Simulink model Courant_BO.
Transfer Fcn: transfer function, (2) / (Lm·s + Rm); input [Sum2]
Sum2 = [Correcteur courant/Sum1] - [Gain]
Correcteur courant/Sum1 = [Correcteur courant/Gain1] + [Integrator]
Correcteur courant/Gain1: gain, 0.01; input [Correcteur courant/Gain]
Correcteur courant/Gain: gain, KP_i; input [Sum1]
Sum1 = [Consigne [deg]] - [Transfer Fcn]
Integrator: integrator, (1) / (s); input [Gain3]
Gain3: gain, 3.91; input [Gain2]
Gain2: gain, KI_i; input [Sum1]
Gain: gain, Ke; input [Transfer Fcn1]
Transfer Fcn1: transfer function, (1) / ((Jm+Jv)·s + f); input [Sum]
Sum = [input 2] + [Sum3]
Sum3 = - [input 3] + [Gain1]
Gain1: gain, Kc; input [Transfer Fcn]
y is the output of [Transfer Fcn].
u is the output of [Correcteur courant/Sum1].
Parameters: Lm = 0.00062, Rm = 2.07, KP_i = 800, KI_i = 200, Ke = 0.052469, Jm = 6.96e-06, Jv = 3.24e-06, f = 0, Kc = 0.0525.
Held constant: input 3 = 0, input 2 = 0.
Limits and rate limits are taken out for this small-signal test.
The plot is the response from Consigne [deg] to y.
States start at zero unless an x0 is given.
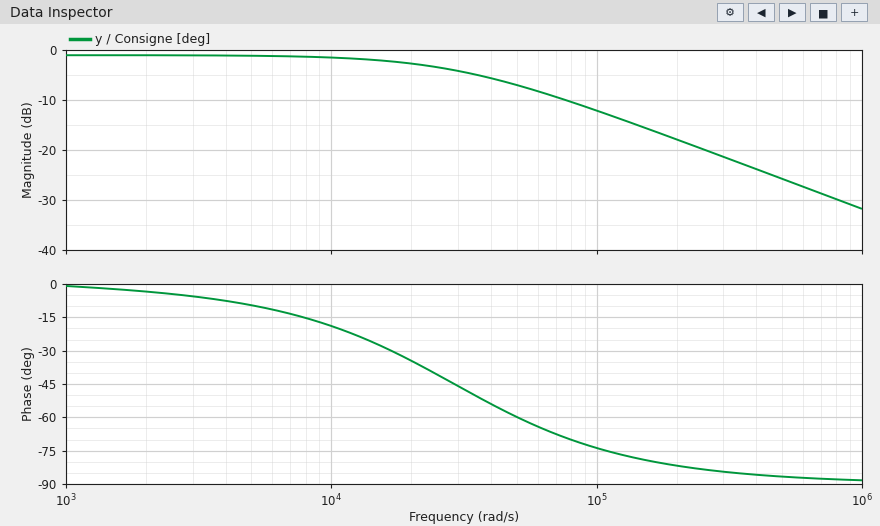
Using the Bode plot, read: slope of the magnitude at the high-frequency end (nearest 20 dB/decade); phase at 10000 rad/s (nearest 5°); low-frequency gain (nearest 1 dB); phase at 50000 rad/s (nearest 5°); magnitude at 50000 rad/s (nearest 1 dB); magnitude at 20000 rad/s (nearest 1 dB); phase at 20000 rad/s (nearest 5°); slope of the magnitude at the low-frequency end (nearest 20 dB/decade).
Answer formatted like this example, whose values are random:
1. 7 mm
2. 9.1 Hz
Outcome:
1. -20 dB/decade
2. -20°
3. -1 dB
4. -60°
5. -7 dB
6. -3 dB
7. -35°
8. 0 dB/decade
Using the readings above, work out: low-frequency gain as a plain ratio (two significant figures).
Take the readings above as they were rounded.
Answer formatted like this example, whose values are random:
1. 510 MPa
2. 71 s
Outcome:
1. 0.89
